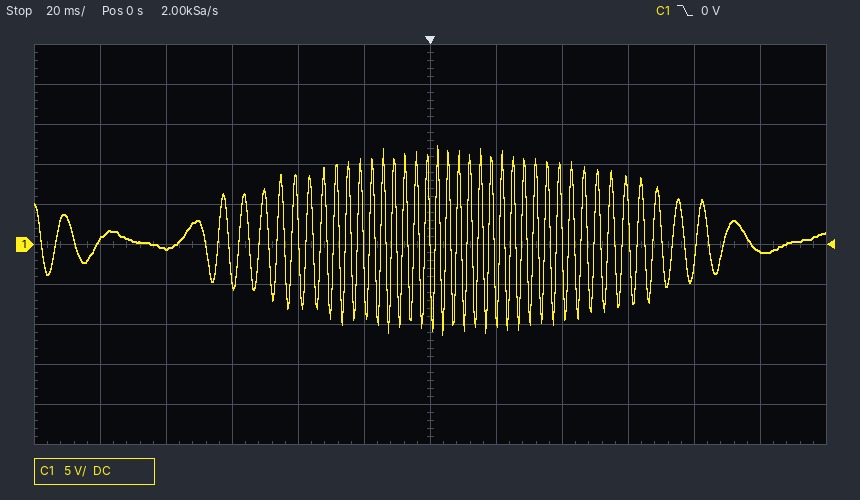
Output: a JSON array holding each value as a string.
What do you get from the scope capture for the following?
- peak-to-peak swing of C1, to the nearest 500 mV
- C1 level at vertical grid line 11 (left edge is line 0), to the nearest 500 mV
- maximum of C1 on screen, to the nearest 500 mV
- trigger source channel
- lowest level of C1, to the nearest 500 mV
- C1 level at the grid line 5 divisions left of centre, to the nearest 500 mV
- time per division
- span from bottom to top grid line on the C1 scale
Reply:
["23.5 V", "-1.0 V", "12.5 V", "C1", "-11.0 V", "500 mV", "20 ms", "50 V"]
